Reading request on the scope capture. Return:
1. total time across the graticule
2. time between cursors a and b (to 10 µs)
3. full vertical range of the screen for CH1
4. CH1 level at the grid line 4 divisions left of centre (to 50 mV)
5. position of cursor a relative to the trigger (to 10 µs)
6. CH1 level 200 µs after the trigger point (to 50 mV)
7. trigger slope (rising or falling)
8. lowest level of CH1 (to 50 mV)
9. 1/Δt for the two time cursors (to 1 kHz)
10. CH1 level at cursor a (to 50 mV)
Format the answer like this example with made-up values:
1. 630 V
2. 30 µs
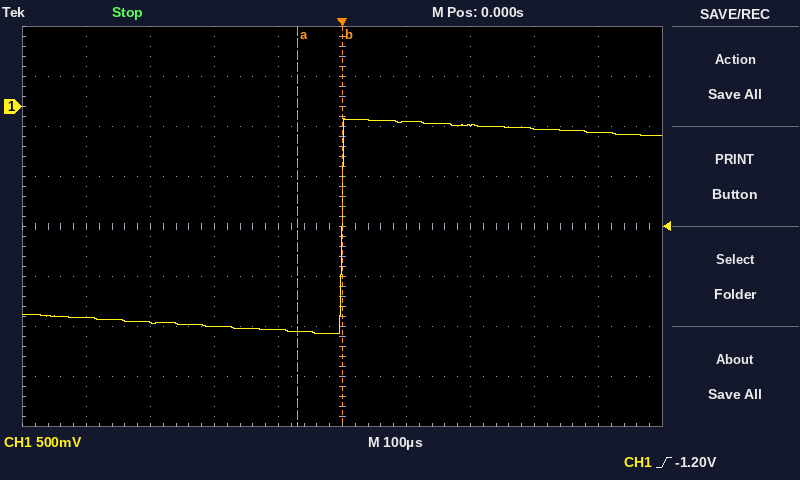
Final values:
1. 1 ms
2. 70 µs
3. 4 V
4. -2.10 V
5. -70 µs
6. -200 mV
7. rising
8. -2.25 V
9. 14 kHz
10. -2.25 V
